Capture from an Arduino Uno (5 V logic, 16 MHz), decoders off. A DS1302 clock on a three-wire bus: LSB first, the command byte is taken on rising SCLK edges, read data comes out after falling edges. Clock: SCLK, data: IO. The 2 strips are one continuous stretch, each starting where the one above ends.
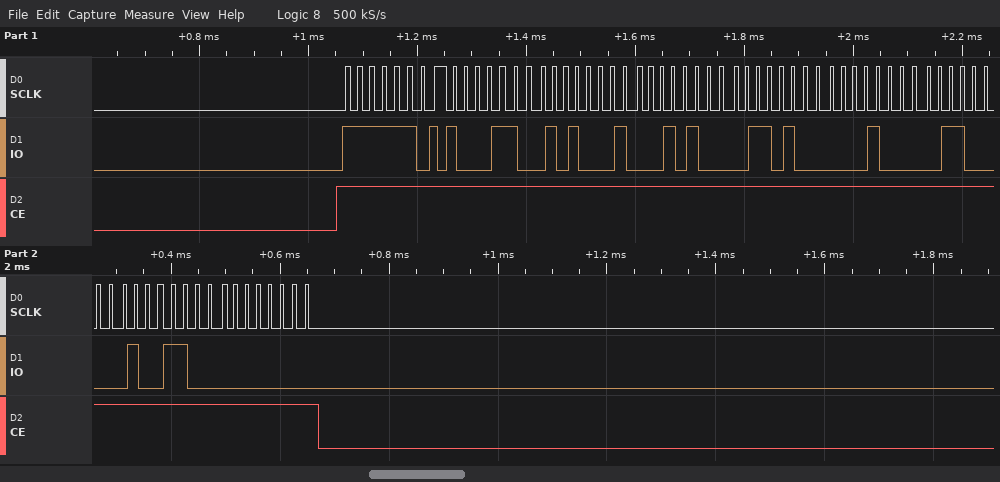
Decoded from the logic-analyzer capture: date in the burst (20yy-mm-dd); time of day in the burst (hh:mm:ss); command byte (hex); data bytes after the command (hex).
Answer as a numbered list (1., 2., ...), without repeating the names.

1. 2019-08-16
2. 14:45:31
3. 0xBF
4. 31 45 14 16 08 06 19 00
